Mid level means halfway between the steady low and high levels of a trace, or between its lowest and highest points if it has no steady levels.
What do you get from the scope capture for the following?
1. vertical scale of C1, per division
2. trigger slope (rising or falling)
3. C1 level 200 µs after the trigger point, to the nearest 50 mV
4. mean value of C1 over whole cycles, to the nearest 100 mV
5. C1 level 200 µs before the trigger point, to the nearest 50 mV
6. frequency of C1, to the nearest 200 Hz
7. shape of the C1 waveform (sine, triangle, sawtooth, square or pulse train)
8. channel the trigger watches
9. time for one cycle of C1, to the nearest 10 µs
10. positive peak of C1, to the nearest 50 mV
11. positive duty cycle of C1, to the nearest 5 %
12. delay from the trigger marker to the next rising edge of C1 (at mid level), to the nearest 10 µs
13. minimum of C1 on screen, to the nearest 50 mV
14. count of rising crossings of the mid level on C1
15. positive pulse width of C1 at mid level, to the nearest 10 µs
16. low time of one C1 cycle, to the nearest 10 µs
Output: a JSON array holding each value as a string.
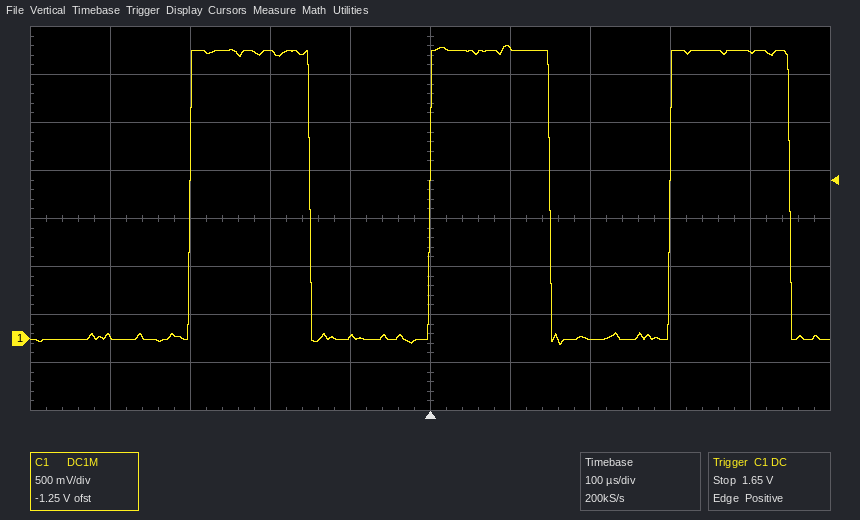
["500 mV", "rising", "0 mV", "1.5 V", "3.00 V", "3.4 kHz", "square", "C1", "300 µs", "3.05 V", "50 %", "300 µs", "-50 mV", "3", "150 µs", "150 µs"]
